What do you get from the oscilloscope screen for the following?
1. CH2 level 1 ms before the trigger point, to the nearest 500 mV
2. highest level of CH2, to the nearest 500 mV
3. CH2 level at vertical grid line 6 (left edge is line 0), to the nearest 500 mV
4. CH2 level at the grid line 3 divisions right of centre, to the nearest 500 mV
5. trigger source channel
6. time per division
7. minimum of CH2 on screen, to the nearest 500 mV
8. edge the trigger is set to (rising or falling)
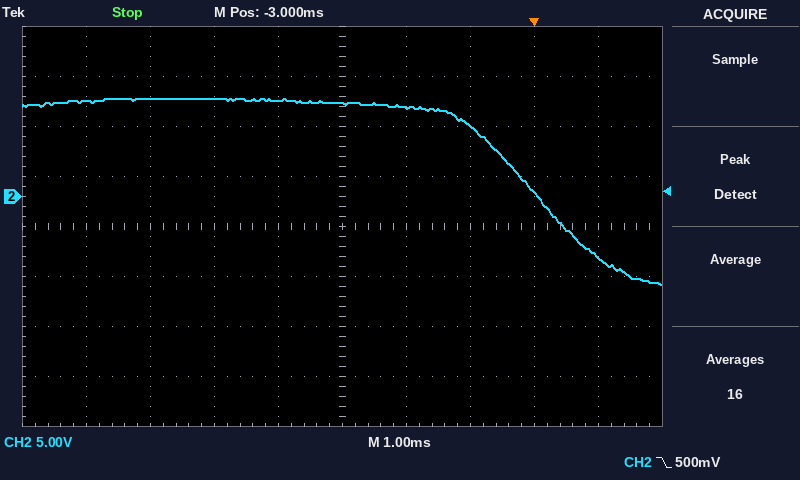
7.0 V
10.0 V
9.0 V
500 mV
CH2
1 ms
-9.0 V
falling
